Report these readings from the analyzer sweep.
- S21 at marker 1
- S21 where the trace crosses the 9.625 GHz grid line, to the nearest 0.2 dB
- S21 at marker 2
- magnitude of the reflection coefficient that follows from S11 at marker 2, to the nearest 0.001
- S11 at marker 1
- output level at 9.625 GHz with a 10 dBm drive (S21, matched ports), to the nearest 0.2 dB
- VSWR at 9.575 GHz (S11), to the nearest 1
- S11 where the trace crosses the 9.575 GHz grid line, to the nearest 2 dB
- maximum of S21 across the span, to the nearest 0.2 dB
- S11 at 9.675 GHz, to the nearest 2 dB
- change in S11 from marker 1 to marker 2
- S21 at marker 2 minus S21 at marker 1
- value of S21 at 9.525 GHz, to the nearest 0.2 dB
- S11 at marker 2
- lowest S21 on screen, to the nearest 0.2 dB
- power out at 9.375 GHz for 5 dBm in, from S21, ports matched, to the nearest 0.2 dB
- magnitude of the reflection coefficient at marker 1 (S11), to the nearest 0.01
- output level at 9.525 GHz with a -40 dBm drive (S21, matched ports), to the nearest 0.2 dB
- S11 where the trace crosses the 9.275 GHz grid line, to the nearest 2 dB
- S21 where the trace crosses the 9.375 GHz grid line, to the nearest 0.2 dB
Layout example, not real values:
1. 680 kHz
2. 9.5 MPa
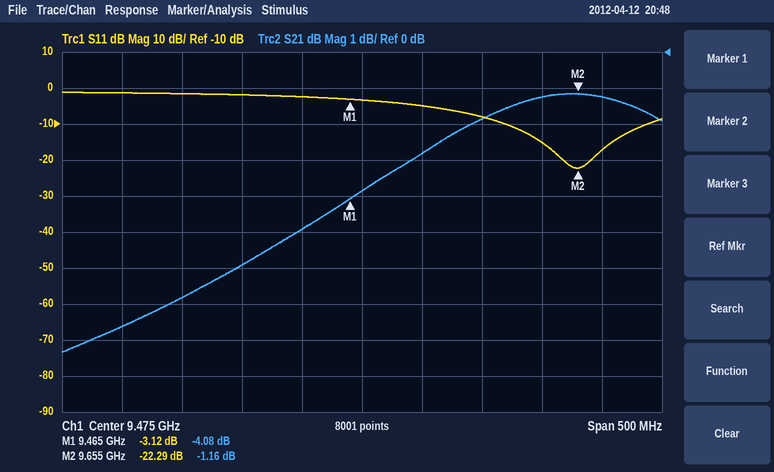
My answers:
1. -4.08 dB
2. -1.2 dB
3. -1.16 dB
4. 0.077
5. -3.12 dB
6. 8.8 dBm
7. 2
8. -8 dB
9. -1.2 dB
10. -18 dB
11. -19.17 dB
12. 2.92 dB
13. -2.8 dB
14. -22.29 dB
15. -8.4 dB
16. -1.0 dBm
17. 0.70
18. -42.8 dBm
19. -2 dB
20. -6.0 dB
